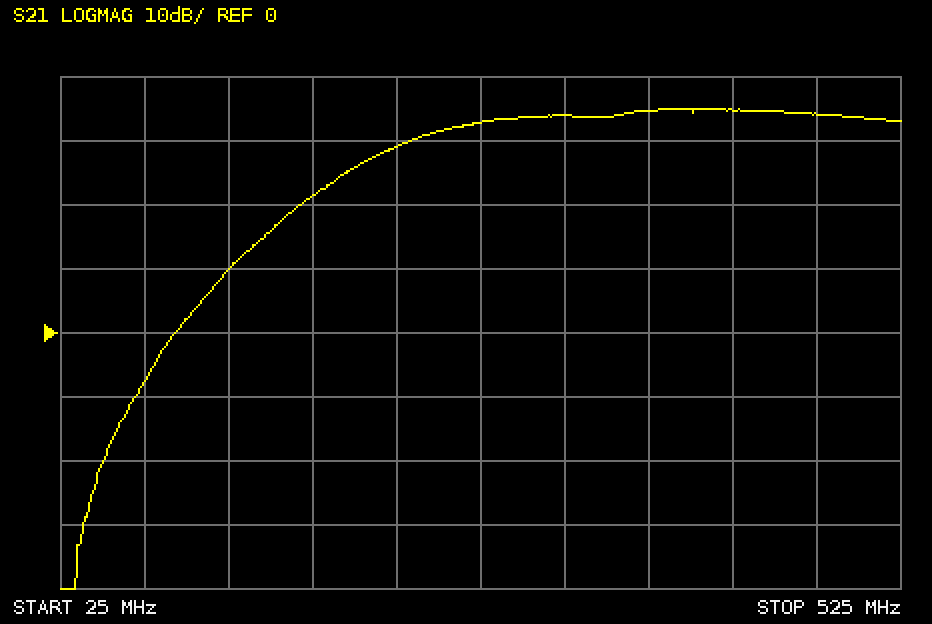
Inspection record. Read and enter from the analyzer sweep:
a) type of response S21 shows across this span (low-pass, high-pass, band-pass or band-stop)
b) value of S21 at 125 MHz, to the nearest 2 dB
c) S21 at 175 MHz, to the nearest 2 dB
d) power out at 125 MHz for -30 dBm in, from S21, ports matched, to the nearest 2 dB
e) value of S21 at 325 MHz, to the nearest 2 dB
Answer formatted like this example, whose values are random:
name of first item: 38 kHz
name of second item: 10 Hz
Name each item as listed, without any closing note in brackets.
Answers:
type of response S21 shows across this span: high-pass
value of S21 at 125 MHz, to the nearest 2 dB: 10 dB
S21 at 175 MHz, to the nearest 2 dB: 22 dB
power out at 125 MHz for -30 dBm in, from S21, ports matched, to the nearest 2 dB: -20 dBm
value of S21 at 325 MHz, to the nearest 2 dB: 34 dB
